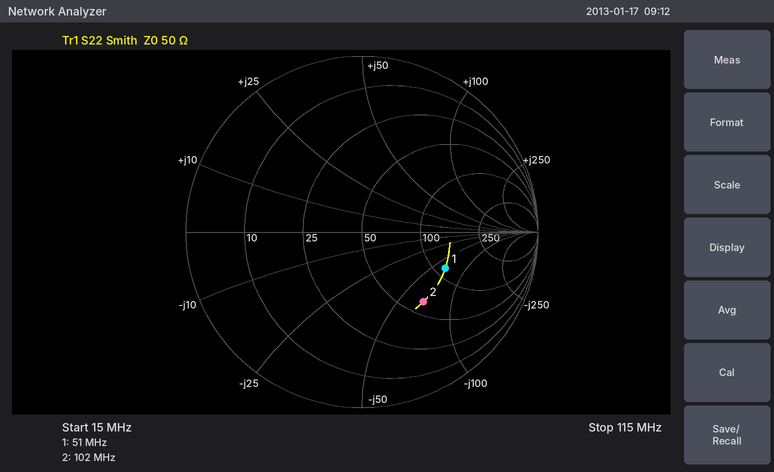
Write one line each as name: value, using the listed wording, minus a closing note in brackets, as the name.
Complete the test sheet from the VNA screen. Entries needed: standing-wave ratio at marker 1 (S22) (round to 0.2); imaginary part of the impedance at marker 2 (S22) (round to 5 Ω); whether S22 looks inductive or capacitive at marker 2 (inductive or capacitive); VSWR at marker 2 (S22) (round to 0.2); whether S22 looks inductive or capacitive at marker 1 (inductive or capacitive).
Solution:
standing-wave ratio at marker 1 (S22): 3.2
imaginary part of the impedance at marker 2 (S22): -70 Ω
whether S22 looks inductive or capacitive at marker 2: capacitive
VSWR at marker 2 (S22): 3.2
whether S22 looks inductive or capacitive at marker 1: capacitive
